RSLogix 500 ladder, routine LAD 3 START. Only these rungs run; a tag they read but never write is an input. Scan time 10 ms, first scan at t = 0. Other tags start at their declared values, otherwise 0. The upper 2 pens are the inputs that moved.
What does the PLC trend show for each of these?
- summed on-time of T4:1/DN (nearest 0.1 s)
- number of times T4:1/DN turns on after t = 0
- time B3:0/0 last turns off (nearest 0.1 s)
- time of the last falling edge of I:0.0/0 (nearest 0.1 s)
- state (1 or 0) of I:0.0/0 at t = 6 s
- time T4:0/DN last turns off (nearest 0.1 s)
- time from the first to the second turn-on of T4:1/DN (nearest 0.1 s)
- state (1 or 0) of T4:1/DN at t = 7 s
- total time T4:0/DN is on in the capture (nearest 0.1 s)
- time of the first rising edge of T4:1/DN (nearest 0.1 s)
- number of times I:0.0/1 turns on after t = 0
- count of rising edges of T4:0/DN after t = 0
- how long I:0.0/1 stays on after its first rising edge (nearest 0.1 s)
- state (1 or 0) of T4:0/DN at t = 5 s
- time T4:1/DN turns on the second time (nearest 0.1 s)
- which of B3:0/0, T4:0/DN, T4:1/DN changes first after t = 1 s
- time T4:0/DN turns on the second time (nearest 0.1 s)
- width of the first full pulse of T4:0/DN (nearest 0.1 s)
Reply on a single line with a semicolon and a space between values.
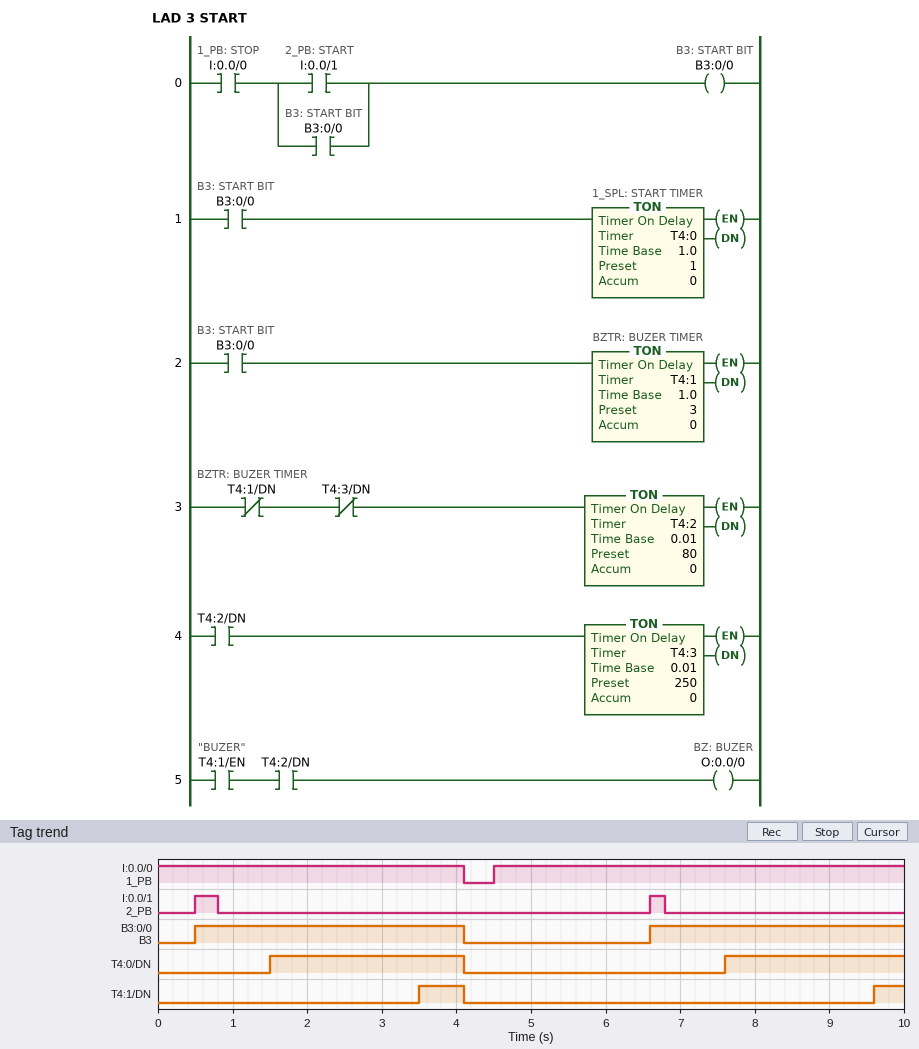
1.0 s; 2; 4.1 s; 4.1 s; 1; 4.1 s; 6.1 s; 0; 5.0 s; 3.5 s; 2; 2; 0.3 s; 0; 9.6 s; T4:0/DN; 7.6 s; 2.6 s
